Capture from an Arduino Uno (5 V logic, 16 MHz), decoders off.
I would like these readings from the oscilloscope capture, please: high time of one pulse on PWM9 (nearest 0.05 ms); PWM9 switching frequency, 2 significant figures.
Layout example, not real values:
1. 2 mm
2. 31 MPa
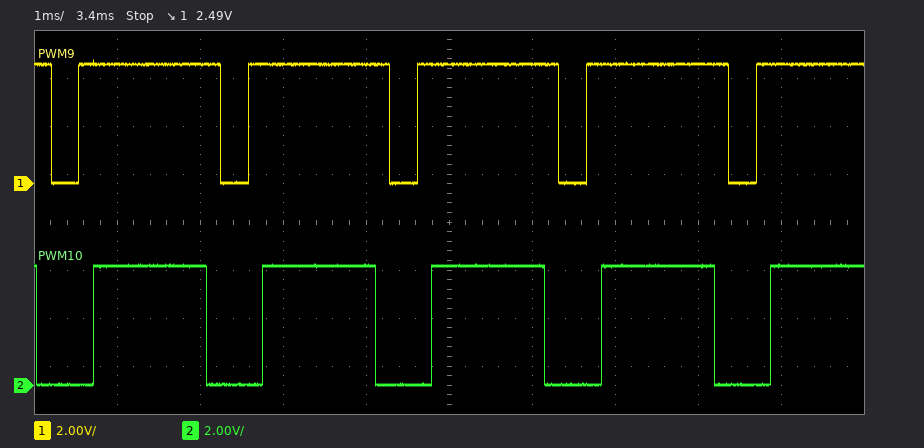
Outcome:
1. 1.70 ms
2. 490 Hz
